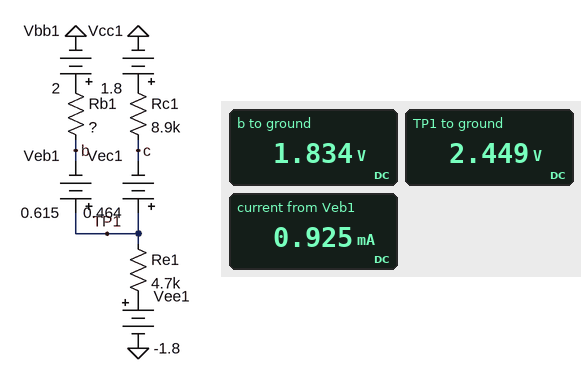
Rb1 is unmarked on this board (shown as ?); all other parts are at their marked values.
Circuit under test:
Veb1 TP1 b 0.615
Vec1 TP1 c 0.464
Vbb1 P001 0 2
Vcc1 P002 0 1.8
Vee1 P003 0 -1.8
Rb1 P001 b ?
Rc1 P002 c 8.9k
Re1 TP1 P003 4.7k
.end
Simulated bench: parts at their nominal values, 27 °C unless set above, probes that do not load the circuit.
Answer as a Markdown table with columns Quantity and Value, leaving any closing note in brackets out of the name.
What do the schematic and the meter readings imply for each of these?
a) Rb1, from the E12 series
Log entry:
| Quantity | Value |
|---|---|
| Rb1, from the E12 series | 180 Ω |
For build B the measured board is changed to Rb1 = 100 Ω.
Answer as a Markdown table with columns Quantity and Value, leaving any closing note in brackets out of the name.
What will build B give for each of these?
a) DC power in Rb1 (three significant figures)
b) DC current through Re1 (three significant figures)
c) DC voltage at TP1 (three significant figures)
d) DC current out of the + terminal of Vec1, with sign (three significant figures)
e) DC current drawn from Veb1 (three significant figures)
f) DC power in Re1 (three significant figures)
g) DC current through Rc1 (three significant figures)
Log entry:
| Quantity | Value |
|---|---|
| DC power in Rb1 | 89.9 µW |
| DC current through Re1 | 919 µA |
| DC voltage at TP1 | 2.52 V |
| DC current out of the + terminal of Vec1, with sign | -28.8 µA |
| DC current drawn from Veb1 | 948 µA |
| DC power in Re1 | 3.97 mW |
| DC current through Rc1 | 28.8 µA |
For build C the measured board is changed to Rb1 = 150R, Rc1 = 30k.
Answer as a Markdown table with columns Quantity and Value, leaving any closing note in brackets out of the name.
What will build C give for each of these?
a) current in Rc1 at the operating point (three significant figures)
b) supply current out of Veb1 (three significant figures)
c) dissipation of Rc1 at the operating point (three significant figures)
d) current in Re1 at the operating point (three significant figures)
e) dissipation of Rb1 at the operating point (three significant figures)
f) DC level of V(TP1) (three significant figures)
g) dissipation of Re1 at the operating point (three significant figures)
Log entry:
| Quantity | Value |
|---|---|
| current in Rc1 at the operating point | 7.11 µA |
| supply current out of Veb1 | 917 µA |
| dissipation of Rc1 at the operating point | 1.52 µW |
| current in Re1 at the operating point | 910 µA |
| dissipation of Rb1 at the operating point | 126 µW |
| DC level of V(TP1) | 2.48 V |
| dissipation of Re1 at the operating point | 3.89 mW |
